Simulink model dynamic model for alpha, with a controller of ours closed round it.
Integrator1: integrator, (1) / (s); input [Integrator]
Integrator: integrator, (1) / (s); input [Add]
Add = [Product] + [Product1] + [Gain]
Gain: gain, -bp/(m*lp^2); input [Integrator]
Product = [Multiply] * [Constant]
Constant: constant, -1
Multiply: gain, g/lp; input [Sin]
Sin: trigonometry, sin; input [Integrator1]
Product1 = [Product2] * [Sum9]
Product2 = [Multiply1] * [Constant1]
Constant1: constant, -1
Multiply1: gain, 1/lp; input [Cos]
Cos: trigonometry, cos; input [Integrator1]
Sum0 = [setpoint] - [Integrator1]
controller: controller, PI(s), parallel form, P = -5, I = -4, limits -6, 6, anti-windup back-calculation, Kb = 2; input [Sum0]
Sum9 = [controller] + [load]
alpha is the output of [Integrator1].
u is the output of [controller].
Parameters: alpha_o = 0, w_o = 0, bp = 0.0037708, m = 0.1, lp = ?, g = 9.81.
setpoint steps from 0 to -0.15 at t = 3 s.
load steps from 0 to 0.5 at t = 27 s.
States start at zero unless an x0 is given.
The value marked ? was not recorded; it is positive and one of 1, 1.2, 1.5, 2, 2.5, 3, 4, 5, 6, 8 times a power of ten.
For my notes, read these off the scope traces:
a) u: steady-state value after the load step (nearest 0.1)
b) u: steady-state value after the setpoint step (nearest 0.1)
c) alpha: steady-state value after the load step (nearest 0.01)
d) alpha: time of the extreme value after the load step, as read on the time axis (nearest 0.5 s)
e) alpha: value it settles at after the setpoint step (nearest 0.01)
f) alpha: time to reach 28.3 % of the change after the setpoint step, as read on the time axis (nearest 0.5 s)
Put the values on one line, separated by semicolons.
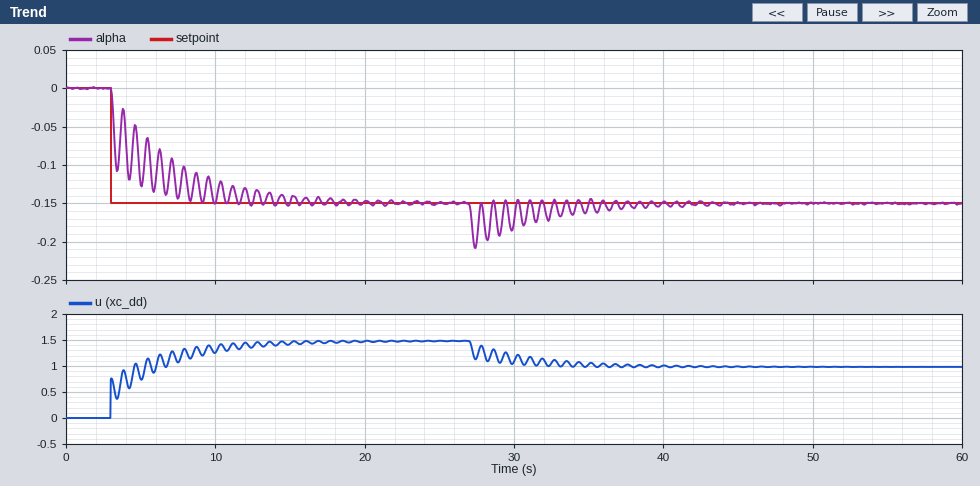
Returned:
1.0; 1.5; -0.15; 27.5 s; -0.15; 3.0 s
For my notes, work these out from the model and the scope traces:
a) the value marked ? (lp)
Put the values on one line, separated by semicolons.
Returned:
0.25
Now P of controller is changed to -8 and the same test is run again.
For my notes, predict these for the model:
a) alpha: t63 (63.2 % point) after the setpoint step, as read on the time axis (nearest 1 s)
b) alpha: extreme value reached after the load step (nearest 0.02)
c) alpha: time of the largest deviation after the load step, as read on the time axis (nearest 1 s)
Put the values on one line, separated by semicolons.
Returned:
3 s; -0.20; 27 s
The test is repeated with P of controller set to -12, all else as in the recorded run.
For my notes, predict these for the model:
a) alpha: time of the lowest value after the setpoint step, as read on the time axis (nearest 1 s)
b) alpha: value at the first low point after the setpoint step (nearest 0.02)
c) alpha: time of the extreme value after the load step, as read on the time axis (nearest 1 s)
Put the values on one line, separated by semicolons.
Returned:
3 s; -0.16; 27 s
